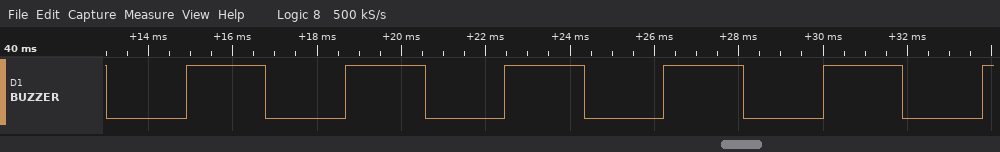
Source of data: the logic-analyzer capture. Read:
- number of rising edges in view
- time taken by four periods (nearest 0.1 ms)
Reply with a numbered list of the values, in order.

1. 6
2. 15.1 ms
